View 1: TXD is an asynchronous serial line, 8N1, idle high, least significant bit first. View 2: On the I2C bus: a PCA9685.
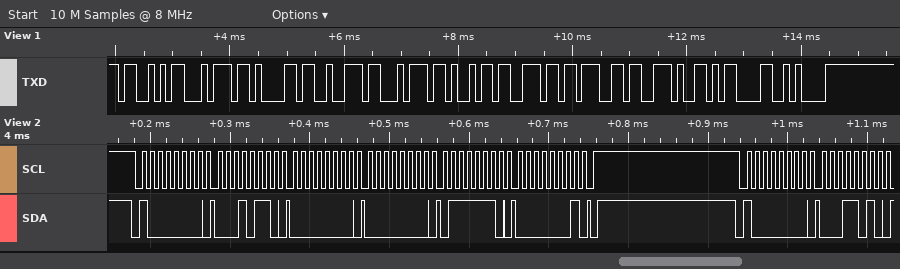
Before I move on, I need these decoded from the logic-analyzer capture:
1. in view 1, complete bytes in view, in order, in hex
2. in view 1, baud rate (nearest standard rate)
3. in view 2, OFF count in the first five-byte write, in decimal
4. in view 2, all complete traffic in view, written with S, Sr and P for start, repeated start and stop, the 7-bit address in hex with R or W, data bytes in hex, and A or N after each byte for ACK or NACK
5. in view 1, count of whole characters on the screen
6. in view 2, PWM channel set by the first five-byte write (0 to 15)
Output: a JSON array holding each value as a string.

["53 74 61 72 74 69 6E 67 2E 0D 0A", "9600 baud", "382", "S 40W A 16 A 00 A 00 A 7E A 01 A P S 40W A 1A A", "11", "4"]
